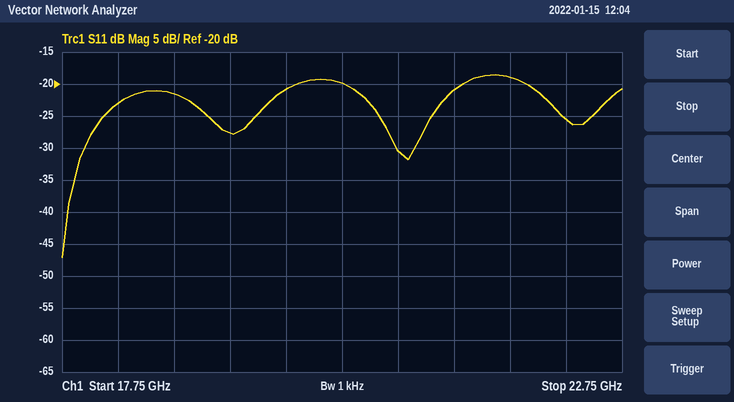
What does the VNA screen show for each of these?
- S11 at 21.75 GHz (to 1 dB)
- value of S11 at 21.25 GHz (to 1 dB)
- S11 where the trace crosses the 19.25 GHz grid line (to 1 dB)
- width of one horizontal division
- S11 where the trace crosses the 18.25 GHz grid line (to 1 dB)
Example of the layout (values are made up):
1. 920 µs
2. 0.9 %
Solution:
1. -19 dB
2. -21 dB
3. -28 dB
4. 500 MHz
5. -23 dB
